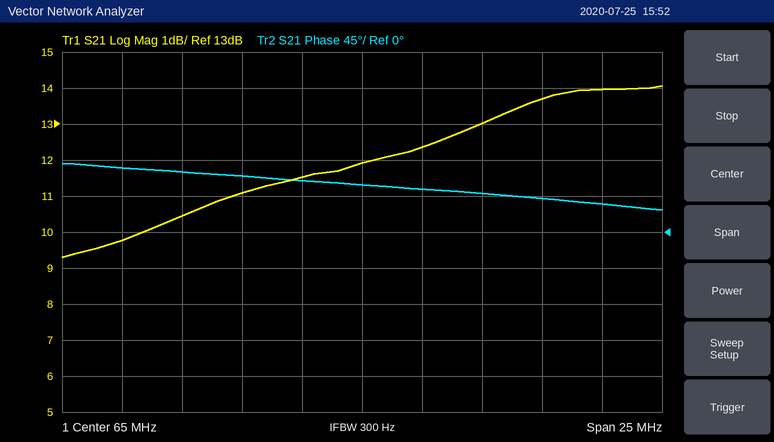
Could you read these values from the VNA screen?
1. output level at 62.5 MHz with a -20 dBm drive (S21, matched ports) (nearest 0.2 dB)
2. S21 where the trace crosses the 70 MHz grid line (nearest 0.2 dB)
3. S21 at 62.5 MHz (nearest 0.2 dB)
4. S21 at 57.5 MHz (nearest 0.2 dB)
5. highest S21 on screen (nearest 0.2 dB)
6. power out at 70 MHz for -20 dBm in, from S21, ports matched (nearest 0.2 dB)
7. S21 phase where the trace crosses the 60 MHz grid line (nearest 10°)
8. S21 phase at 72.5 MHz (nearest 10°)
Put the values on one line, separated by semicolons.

-8.4 dBm; 13.0 dB; 11.6 dB; 10.4 dB; 14.0 dB; -7.0 dBm; 70°; 40°
